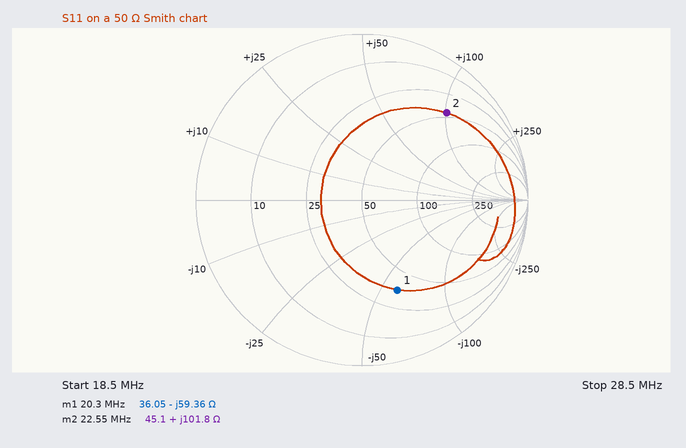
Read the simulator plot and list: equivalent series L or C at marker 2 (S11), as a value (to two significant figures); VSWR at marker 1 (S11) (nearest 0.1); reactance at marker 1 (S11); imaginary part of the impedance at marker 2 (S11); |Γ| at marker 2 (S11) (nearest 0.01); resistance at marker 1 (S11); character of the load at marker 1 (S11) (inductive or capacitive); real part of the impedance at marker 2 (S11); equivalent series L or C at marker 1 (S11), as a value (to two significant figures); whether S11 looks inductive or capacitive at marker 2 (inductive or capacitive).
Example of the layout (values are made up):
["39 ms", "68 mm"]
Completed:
["720 nH", "3.8", "-59.36 Ω", "+101.8 Ω", "0.73", "36.05 Ω", "capacitive", "45.1 Ω", "130 pF", "inductive"]
